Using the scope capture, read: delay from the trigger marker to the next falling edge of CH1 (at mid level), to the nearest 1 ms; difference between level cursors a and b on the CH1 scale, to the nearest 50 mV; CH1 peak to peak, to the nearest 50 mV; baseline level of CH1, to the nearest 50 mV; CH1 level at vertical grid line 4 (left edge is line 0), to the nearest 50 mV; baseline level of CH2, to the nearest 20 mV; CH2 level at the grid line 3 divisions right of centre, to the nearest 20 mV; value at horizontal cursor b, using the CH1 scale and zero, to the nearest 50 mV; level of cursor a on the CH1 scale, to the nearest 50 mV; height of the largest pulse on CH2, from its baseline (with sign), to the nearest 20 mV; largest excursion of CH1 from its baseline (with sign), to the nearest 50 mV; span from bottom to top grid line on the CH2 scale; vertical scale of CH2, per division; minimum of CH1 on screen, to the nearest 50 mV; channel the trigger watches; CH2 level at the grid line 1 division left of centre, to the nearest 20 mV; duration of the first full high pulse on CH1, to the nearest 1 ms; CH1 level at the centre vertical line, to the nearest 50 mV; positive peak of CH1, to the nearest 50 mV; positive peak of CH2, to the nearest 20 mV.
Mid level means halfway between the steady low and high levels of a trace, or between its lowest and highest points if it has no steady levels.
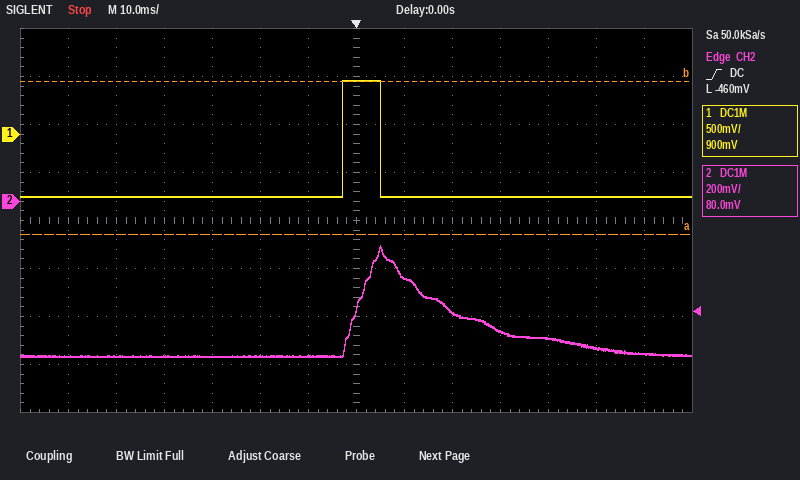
5 ms
1.60 V
1.20 V
-650 mV
-650 mV
-640 mV
-540 mV
550 mV
-1.05 V
+460 mV
+1.20 V
1.6 V
200 mV
-650 mV
CH2
-640 mV
8 ms
550 mV
550 mV
-180 mV
